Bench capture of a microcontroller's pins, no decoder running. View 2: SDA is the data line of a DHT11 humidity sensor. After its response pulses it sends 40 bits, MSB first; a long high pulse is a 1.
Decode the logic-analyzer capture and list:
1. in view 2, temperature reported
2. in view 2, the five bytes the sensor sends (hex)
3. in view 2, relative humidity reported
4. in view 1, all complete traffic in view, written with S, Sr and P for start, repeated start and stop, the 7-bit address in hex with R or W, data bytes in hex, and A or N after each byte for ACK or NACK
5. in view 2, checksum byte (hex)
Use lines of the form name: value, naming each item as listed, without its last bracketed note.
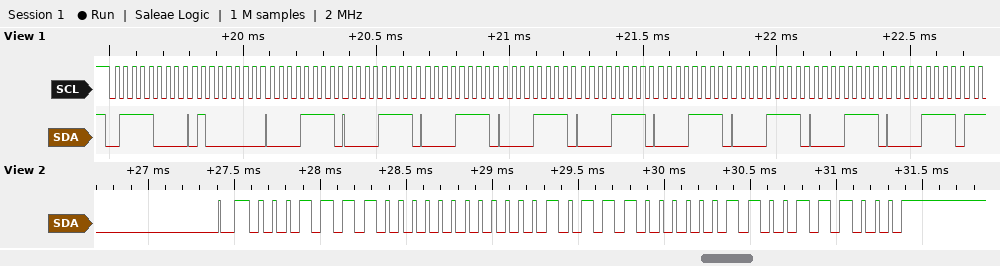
in view 2, temperature reported: 23.3 °C
in view 2, the five bytes the sensor sends: 1E 00 17 03 38
in view 2, relative humidity reported: 30 %
in view 1, all complete traffic in view, written with S, Sr and P for start, repeated start and stop, the 7-bit address in hex with R or W, data bytes in hex, and A or N after each byte for ACK or NACK: S 3CW A 40 A 0F A 0F A 0F A 0F A 0F A 0F A 0F A 0F A 0F A
in view 2, checksum byte: 0x38
